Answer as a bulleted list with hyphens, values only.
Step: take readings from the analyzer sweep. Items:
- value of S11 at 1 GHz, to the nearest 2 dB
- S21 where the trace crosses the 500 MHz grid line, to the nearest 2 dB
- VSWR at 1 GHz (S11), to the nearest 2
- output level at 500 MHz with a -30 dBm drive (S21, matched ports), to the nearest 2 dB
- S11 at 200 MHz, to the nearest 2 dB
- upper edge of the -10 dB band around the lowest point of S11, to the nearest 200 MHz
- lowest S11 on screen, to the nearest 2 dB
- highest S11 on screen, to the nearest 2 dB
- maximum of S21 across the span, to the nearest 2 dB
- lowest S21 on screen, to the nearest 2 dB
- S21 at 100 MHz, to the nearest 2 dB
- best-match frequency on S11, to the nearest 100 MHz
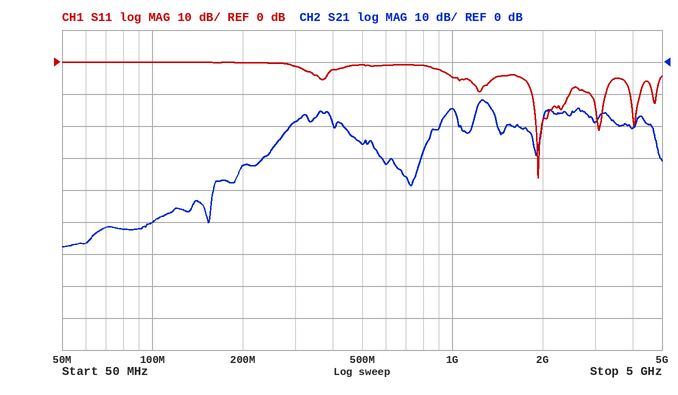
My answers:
- -4 dB
- -26 dB
- 4
- -56 dBm
- 0 dB
- 2.4 GHz
- -36 dB
- 0 dB
- -12 dB
- -58 dB
- -50 dB
- 1.9 GHz
